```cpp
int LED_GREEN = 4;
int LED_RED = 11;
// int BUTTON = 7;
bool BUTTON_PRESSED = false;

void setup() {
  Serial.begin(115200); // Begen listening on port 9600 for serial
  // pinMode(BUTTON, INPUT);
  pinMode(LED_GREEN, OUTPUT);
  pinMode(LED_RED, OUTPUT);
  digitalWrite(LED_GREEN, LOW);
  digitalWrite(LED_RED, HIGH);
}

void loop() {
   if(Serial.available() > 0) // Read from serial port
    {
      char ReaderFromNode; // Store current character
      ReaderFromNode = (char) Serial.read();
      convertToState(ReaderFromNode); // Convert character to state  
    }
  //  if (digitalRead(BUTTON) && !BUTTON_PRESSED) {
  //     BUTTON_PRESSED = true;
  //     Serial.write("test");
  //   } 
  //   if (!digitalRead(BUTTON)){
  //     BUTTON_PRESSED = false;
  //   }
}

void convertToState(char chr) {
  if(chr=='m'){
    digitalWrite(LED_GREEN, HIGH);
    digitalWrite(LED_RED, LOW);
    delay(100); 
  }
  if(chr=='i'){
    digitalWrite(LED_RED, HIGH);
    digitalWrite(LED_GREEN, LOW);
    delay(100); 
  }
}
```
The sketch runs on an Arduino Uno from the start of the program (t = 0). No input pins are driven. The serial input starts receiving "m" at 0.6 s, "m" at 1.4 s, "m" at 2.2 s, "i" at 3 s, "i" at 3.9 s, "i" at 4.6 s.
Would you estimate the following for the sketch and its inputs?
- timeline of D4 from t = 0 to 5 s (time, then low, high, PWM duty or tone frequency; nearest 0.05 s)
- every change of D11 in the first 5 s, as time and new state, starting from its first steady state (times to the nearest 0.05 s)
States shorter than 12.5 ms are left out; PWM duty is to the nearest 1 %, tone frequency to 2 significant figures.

0 s low; 0.6 s high; 3 s low
0 s high; 0.6 s low; 3 s high
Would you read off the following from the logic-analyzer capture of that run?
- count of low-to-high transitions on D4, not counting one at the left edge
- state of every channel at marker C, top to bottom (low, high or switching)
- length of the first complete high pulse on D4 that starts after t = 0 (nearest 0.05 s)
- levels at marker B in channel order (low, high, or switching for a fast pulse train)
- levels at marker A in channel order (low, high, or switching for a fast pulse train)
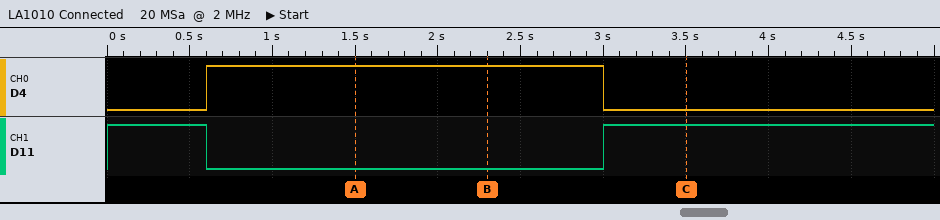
1
D4 low, D11 high
2.40 s
D4 high, D11 low
D4 high, D11 low
